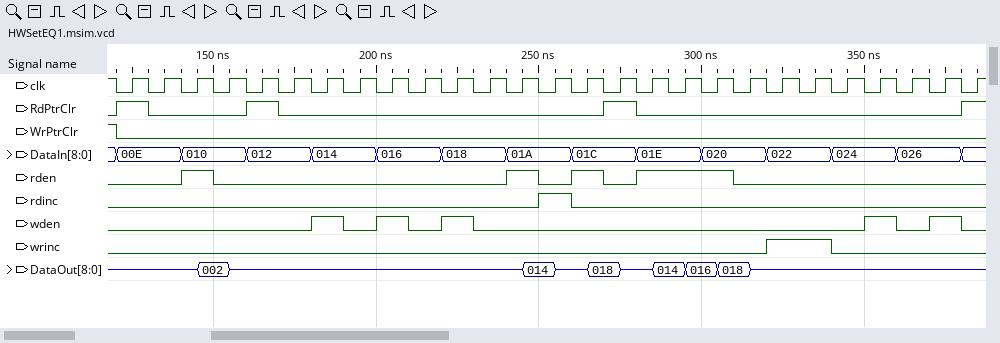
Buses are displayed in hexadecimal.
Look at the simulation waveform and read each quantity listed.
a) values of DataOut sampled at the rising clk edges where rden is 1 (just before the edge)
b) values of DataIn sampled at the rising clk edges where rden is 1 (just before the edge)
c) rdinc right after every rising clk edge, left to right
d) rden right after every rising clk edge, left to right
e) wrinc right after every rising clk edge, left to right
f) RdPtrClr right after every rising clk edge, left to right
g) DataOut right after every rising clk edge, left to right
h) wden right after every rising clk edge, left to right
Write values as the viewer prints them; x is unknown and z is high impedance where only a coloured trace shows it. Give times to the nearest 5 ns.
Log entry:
z, z, z, z, 014, 016
010, 01A, 01C, 01E, 01E, 020
0 0 0 0 0 0 0 0 0 0 0 0 0 1 0 0 0 0 0 0 0 0 0 0 0 0 0
0 0 1 0 0 0 0 0 0 0 0 0 1 0 1 0 1 1 1 0 0 0 0 0 0 0 0
0 0 0 0 0 0 0 0 0 0 0 0 0 0 0 0 0 0 0 0 1 1 0 0 0 0 0
1 0 0 0 1 0 0 0 0 0 0 0 0 0 0 1 0 0 0 0 0 0 0 0 0 0 1
z, z, 002, z, z, z, z, z, z, z, z, z, 014, z, 018, z, 014, 016, 018, z, z, z, z, z, z, z, z
0 0 0 0 0 0 1 0 1 0 1 0 0 0 0 0 0 0 0 0 0 0 0 1 0 1 0
